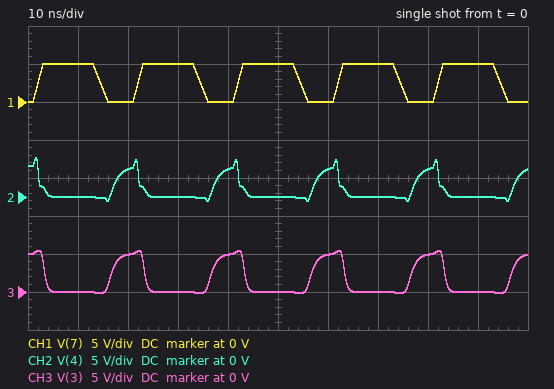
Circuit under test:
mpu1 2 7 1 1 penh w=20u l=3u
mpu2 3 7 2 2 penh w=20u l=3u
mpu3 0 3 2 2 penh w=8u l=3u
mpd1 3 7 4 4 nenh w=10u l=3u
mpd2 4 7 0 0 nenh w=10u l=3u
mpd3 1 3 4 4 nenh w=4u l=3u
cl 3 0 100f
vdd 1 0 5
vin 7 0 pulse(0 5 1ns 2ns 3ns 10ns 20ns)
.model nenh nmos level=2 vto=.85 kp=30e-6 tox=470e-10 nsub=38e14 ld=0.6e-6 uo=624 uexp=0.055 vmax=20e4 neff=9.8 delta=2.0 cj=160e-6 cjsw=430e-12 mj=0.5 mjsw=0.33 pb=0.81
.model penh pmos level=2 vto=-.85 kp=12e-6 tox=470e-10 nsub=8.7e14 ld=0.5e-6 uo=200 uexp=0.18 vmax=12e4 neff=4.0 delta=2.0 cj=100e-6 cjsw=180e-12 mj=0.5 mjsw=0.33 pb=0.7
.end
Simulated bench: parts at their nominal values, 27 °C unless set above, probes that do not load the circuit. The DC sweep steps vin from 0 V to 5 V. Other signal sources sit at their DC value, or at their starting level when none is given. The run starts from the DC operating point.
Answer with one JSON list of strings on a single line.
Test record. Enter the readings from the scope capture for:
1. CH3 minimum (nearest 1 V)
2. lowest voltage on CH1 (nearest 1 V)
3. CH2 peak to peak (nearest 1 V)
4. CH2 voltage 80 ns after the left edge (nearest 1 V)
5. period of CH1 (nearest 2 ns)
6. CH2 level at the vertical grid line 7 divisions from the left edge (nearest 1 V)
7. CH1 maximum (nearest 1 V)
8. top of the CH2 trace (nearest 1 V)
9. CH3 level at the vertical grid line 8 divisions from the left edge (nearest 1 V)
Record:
["0 V", "0 V", "6 V", "4 V", "20 ns", "0 V", "5 V", "5 V", "5 V"]
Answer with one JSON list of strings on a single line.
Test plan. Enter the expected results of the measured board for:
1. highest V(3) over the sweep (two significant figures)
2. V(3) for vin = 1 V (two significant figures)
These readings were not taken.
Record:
["5.0 V", "5.0 V"]
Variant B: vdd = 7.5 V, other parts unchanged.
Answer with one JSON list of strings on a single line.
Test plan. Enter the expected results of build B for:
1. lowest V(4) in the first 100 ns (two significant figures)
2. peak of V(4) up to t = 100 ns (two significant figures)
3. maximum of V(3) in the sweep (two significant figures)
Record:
["-49 mV", "7.7 V", "7.5 V"]
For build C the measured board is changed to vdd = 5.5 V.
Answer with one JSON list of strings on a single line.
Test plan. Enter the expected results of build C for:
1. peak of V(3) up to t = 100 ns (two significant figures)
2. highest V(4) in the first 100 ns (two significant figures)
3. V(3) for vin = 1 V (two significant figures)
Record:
["5.9 V", "5.7 V", "5.5 V"]
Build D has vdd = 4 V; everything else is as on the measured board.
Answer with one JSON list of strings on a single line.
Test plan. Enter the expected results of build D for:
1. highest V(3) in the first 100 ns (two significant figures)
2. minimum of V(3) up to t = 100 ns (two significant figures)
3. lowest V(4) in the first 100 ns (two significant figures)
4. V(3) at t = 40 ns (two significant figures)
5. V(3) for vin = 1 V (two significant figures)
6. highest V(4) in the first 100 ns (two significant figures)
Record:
["4.4 V", "-170 mV", "-560 mV", "3.7 V", "4.0 V", "4.2 V"]
